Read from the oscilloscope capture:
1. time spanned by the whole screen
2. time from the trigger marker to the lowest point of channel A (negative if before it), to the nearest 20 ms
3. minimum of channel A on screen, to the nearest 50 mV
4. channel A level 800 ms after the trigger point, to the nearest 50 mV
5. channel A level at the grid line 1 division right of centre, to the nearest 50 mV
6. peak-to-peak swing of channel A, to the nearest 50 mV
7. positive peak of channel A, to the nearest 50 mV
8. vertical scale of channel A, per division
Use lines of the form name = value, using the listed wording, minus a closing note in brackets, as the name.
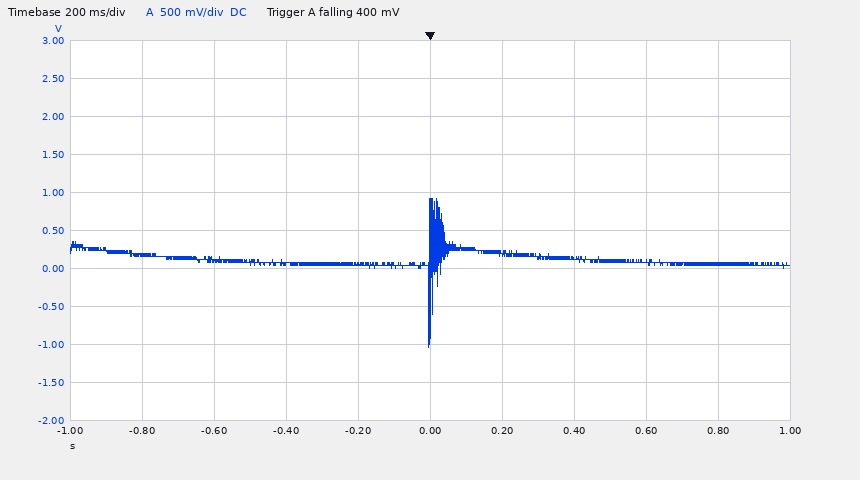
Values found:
time spanned by the whole screen = 2 s
time from the trigger marker to the lowest point of channel A (negative if before it), to the nearest 20 ms = 0 ms
minimum of channel A on screen, to the nearest 50 mV = -1.05 V
channel A level 800 ms after the trigger point, to the nearest 50 mV = 50 mV
channel A level at the grid line 1 division right of centre, to the nearest 50 mV = 200 mV
peak-to-peak swing of channel A, to the nearest 50 mV = 1.95 V
positive peak of channel A, to the nearest 50 mV = 900 mV
vertical scale of channel A, per division = 500 mV
